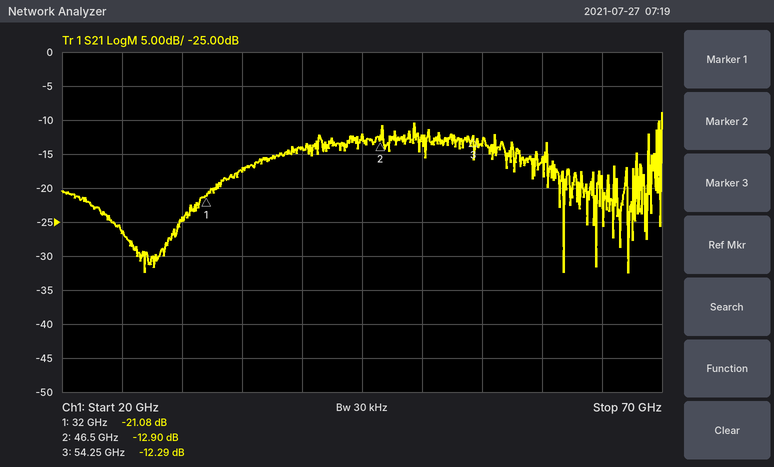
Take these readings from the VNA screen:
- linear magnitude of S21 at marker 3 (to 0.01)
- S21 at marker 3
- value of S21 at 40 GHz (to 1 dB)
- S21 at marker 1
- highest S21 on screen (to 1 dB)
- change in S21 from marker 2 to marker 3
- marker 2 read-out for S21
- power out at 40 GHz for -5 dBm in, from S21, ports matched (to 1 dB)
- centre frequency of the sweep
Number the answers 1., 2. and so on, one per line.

1. 0.24
2. -12.29 dB
3. -14 dB
4. -21.08 dB
5. -9 dB
6. 0.61 dB
7. -12.90 dB
8. -19 dBm
9. 45 GHz
